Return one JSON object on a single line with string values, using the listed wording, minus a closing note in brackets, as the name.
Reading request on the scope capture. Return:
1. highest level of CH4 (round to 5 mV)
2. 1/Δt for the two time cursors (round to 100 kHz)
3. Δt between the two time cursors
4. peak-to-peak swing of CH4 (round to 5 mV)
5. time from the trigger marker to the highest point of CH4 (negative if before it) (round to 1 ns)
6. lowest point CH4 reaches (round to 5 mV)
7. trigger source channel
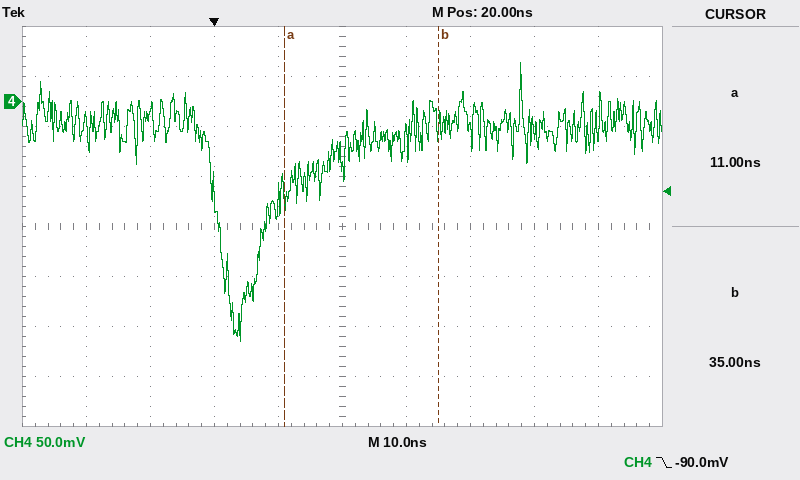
{"highest level of CH4": "40 mV", "1/Δt for the two time cursors": "41.7 MHz", "Δt between the two time cursors": "24 ns", "peak-to-peak swing of CH4": "280 mV", "time from the trigger marker to the highest point of CH4 (negative if before it)": "+48 ns", "lowest point CH4 reaches": "-240 mV", "trigger source channel": "CH4"}
